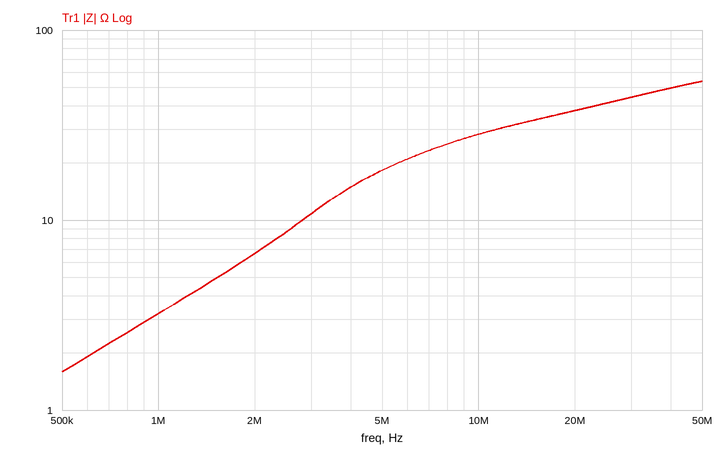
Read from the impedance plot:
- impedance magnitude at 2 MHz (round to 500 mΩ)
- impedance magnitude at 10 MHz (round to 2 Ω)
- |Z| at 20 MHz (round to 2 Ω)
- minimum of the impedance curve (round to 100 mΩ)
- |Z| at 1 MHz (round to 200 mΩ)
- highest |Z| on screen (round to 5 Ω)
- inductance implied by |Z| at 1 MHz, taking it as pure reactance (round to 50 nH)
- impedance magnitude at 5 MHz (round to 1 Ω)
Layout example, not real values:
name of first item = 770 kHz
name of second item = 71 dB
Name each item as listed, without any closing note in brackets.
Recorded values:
impedance magnitude at 2 MHz = 6.5 Ω
impedance magnitude at 10 MHz = 28 Ω
|Z| at 20 MHz = 38 Ω
minimum of the impedance curve = 1.6 Ω
|Z| at 1 MHz = 3.2 Ω
highest |Z| on screen = 55 Ω
inductance implied by |Z| at 1 MHz, taking it as pure reactance = 500 nH
impedance magnitude at 5 MHz = 18 Ω
